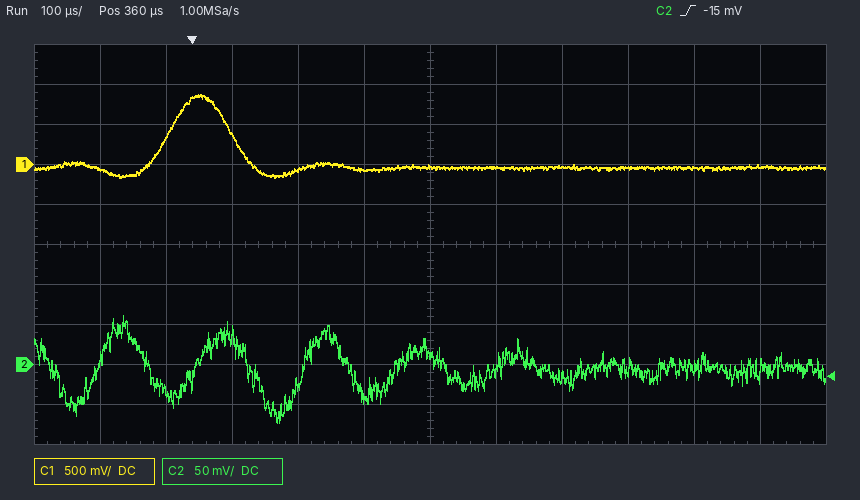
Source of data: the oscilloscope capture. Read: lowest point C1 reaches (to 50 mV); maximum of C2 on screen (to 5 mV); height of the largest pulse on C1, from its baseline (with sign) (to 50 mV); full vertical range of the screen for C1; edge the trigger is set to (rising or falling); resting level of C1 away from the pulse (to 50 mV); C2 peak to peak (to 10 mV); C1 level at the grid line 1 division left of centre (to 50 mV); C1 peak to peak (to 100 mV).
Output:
-150 mV
60 mV
+900 mV
5 V
rising
-50 mV
130 mV
-50 mV
1.00 V
